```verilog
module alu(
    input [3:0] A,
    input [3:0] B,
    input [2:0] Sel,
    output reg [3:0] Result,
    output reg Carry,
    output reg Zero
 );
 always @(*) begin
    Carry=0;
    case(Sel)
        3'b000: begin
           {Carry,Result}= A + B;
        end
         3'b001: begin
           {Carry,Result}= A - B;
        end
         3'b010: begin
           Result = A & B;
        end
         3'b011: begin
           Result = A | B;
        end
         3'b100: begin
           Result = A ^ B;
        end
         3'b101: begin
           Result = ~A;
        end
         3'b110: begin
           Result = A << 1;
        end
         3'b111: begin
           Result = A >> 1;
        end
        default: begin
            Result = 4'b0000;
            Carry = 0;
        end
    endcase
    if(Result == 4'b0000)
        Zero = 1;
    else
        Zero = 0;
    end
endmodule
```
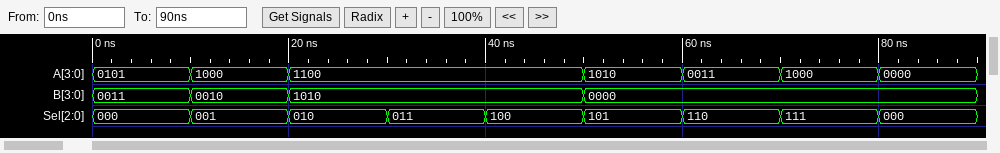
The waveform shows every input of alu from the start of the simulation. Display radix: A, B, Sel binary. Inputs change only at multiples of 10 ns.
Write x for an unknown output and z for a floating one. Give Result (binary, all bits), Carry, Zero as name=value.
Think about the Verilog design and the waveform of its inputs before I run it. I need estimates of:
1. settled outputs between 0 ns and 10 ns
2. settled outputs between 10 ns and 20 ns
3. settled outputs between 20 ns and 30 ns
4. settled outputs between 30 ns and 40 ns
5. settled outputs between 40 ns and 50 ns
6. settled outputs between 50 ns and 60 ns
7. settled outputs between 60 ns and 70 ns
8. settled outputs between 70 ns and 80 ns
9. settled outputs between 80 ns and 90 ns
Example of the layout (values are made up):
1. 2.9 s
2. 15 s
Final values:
1. Result=1000, Carry=0, Zero=0
2. Result=0110, Carry=0, Zero=0
3. Result=1000, Carry=0, Zero=0
4. Result=1110, Carry=0, Zero=0
5. Result=0110, Carry=0, Zero=0
6. Result=0101, Carry=0, Zero=0
7. Result=0110, Carry=0, Zero=0
8. Result=0100, Carry=0, Zero=0
9. Result=0000, Carry=0, Zero=1
